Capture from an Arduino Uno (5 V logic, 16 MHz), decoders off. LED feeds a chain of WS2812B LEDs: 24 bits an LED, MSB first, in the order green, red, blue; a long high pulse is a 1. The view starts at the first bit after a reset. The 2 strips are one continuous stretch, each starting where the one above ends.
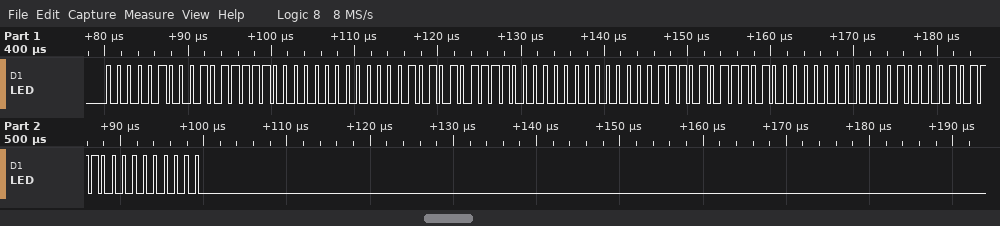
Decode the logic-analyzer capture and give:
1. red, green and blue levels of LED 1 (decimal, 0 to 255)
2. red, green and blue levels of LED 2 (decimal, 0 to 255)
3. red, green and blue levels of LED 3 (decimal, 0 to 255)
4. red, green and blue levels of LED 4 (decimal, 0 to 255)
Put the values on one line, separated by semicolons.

95, 4, 0; 94, 5, 0; 93, 7, 0; 92, 8, 0
